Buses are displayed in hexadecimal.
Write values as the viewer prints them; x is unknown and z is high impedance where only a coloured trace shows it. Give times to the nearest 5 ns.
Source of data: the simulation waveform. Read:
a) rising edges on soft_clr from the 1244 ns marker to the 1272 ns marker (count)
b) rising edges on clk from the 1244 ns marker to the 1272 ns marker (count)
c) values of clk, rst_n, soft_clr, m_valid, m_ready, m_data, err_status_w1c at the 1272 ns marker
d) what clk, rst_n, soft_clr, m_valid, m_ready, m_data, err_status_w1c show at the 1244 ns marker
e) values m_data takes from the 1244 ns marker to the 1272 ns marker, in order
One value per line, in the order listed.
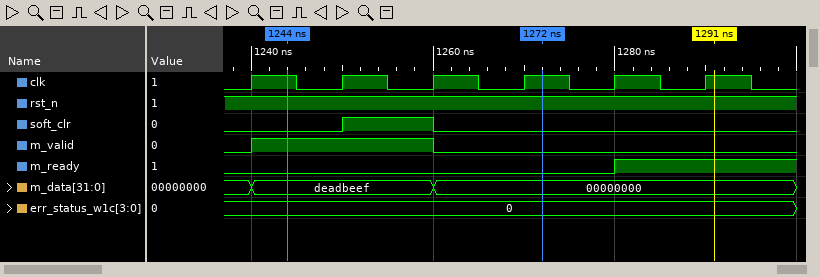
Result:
1
3
clk=1, rst_n=1, soft_clr=0, m_valid=0, m_ready=0, m_data=00000000, err_status_w1c=0
clk=1, rst_n=1, soft_clr=0, m_valid=1, m_ready=0, m_data=deadbeef, err_status_w1c=0
deadbeef, 00000000
